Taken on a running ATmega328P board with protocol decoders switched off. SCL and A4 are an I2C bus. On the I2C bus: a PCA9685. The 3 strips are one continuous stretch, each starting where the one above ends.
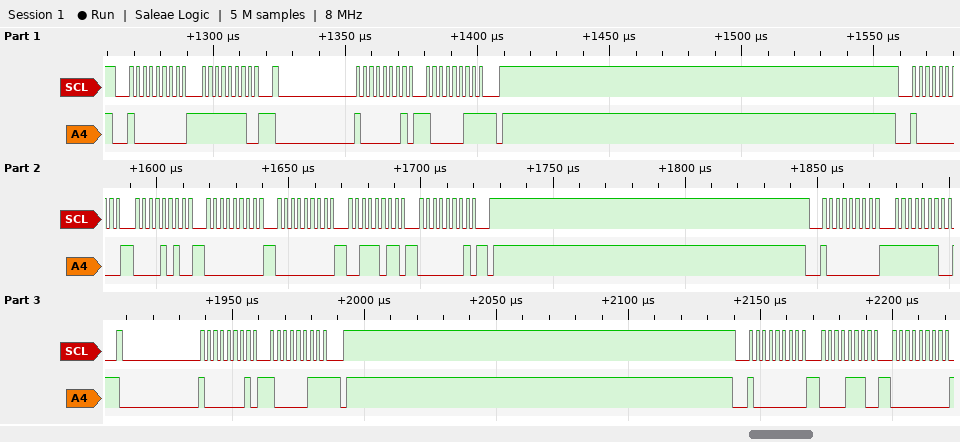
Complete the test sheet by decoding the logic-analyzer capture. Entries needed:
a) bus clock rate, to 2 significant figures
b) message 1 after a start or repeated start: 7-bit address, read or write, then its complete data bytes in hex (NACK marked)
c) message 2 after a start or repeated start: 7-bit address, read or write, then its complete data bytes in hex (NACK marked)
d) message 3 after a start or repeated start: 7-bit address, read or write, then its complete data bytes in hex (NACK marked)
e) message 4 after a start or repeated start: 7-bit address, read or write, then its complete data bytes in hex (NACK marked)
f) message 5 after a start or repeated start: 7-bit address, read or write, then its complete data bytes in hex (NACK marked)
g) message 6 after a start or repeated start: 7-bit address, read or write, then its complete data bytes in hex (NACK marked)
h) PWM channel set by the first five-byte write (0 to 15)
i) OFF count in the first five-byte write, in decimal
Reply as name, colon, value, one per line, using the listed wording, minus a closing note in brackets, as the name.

bus clock rate, to 2 significant figures: 400 kHz
message 1 after a start or repeated start: 7-bit address, read or write, then its complete data bytes in hex: 0x40 write: FE
message 2 after a start or repeated start: 7-bit address, read or write, then its complete data bytes in hex: 0x40 read: 83 NACK
message 3 after a start or repeated start: 7-bit address, read or write, then its complete data bytes in hex: 0x40 write: 0A 00 00 3B 01
message 4 after a start or repeated start: 7-bit address, read or write, then its complete data bytes in hex: 0x40 write: FE
message 5 after a start or repeated start: 7-bit address, read or write, then its complete data bytes in hex: 0x40 read: 83 NACK
message 6 after a start or repeated start: 7-bit address, read or write, then its complete data bytes in hex: 0x40 write: 0E 00
PWM channel set by the first five-byte write: 1
OFF count in the first five-byte write, in decimal: 315
